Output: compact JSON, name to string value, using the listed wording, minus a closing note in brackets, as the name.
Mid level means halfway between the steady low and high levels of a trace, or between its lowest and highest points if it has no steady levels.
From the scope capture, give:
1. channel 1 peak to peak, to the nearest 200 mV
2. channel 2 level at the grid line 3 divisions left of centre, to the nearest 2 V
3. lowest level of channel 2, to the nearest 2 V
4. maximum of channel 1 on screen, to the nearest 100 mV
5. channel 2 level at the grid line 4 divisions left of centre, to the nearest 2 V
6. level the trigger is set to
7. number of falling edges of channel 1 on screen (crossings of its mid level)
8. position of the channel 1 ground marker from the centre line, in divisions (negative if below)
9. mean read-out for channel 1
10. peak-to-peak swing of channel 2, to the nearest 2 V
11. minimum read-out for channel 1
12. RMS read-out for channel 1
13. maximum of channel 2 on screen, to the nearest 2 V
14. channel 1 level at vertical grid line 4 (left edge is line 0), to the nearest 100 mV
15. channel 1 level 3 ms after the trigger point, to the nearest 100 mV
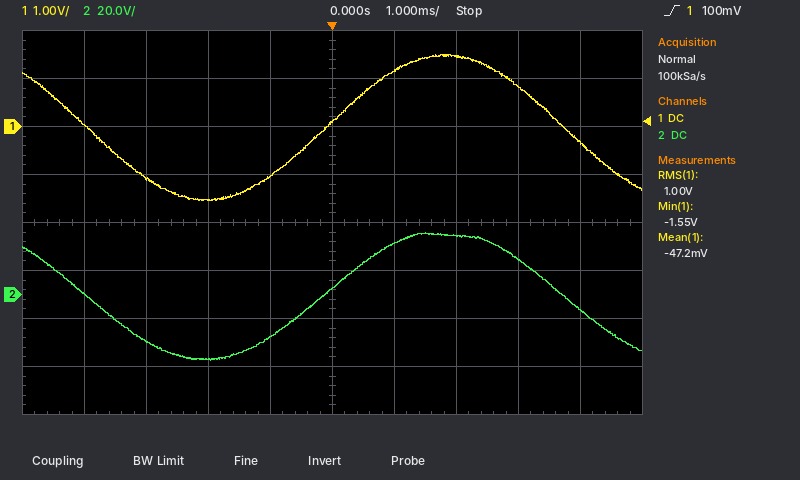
{"channel 1 peak to peak, to the nearest 200 mV": "3.0 V", "channel 2 level at the grid line 3 divisions left of centre, to the nearest 2 V": "-20 V", "lowest level of channel 2, to the nearest 2 V": "-28 V", "maximum of channel 1 on screen, to the nearest 100 mV": "1.5 V", "channel 2 level at the grid line 4 divisions left of centre, to the nearest 2 V": "0 V", "level the trigger is set to": "100 mV", "number of falling edges of channel 1 on screen": "2", "position of the channel 1 ground marker from the centre line, in divisions": "+2.0 div", "mean read-out for channel 1": "-47.2 mV", "peak-to-peak swing of channel 2, to the nearest 2 V": "54 V", "minimum read-out for channel 1": "-1.55 V", "RMS read-out for channel 1": "1.00 V", "maximum of channel 2 on screen, to the nearest 2 V": "26 V", "channel 1 level at vertical grid line 4 (left edge is line 0), to the nearest 100 mV": "-1.0 V", "channel 1 level 3 ms after the trigger point, to the nearest 100 mV": "800 mV"}
